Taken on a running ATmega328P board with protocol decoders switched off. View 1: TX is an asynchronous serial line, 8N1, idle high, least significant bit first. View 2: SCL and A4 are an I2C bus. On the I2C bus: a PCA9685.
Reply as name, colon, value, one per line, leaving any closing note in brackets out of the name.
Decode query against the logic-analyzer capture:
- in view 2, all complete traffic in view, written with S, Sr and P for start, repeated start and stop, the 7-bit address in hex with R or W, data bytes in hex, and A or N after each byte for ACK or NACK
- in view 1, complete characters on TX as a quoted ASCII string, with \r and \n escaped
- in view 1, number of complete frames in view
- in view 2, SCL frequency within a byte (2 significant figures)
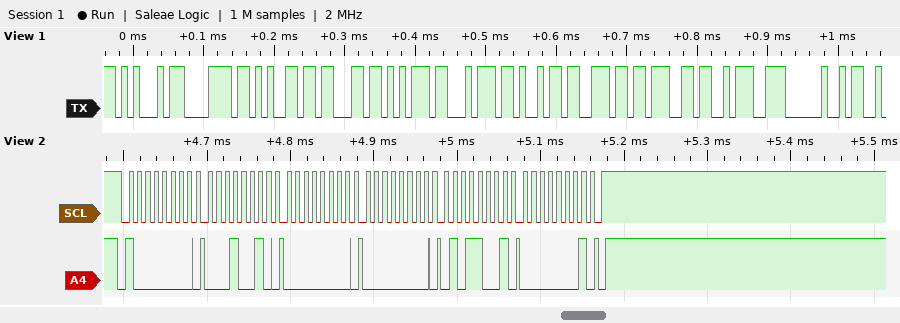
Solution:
in view 2, all complete traffic in view, written with S, Sr and P for start, repeated start and stop, the 7-bit address in hex with R or W, data bytes in hex, and A or N after each byte for ACK or NACK: S 40W A 12 A 00 A 00 A 59 A 01 A P
in view 1, complete characters on TX as a quoted ASCII string, with \r and \n escaped: "Executing: "
in view 1, number of complete frames in view: 11
in view 2, SCL frequency within a byte: 100 kHz
